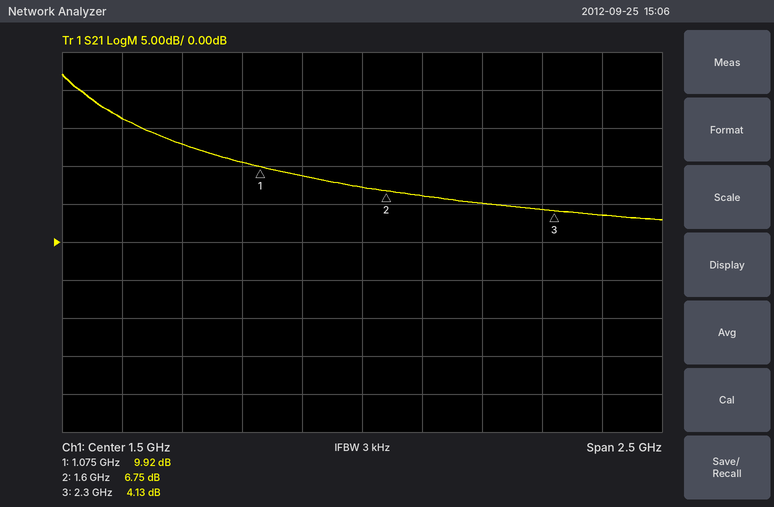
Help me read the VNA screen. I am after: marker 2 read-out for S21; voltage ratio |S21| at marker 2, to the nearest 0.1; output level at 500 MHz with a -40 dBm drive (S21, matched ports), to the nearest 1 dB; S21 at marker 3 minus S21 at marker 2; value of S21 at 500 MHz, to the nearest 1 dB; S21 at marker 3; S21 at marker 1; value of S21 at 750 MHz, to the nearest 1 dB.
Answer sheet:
6.75 dB
2.2
-24 dBm
-2.62 dB
16 dB
4.13 dB
9.92 dB
13 dB
